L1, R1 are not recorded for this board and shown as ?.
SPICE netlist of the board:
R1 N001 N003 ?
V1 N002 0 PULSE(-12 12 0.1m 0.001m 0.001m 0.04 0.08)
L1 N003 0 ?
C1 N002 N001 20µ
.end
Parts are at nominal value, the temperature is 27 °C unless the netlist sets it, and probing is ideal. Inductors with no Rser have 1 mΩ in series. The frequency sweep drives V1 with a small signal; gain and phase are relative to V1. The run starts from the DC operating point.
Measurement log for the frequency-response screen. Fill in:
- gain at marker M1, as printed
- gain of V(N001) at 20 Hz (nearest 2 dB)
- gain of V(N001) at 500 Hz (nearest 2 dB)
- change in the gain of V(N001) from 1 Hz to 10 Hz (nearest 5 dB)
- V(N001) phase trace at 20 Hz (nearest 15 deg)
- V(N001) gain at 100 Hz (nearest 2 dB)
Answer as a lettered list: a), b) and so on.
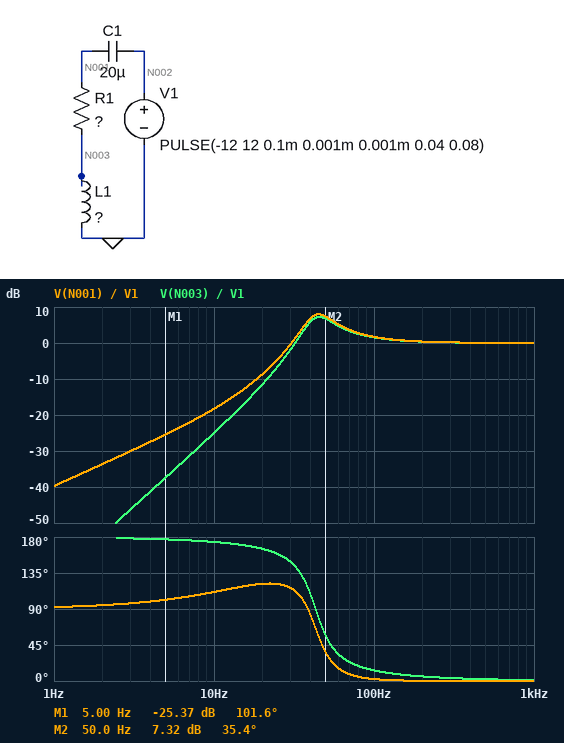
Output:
a) -25.37 dB
b) -8 dB
c) 0 dB
d) 20 dB
e) 120 deg
f) 2 dB
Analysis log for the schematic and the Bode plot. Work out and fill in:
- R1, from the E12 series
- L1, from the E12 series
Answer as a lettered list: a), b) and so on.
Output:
a) 82 Ω
b) 680 mH
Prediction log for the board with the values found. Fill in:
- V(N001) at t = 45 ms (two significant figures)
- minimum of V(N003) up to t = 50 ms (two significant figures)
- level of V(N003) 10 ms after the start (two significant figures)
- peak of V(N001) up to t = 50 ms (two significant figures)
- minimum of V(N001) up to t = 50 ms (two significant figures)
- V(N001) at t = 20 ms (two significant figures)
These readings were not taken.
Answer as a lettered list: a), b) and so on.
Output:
a) -7.8 V
b) -24 V
c) -13 V
d) 24 V
e) -25 V
f) 2.4 V
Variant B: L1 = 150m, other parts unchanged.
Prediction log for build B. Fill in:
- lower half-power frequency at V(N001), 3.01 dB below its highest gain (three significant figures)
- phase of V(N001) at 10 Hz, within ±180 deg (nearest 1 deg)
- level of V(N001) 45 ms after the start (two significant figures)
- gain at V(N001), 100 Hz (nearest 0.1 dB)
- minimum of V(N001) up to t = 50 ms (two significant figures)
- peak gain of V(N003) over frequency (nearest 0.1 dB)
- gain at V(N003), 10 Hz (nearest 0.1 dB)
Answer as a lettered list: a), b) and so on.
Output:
a) 68.0 Hz
b) 91 deg
c) 3.0 V
d) 3.5 dB
e) -24 V
f) 1.6 dB
g) -38.5 dB
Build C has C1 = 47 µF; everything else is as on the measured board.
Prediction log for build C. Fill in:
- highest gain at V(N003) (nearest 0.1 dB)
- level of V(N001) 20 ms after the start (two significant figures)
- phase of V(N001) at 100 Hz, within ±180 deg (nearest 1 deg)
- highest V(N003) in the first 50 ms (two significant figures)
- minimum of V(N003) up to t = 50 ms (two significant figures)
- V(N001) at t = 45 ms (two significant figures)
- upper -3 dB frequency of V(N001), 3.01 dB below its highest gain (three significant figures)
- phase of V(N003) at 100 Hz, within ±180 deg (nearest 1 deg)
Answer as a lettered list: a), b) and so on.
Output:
a) 3.9 dB
b) -7.6 V
c) 1 deg
d) 24 V
e) -22 V
f) -16 V
g) 55.4 Hz
h) 12 deg
